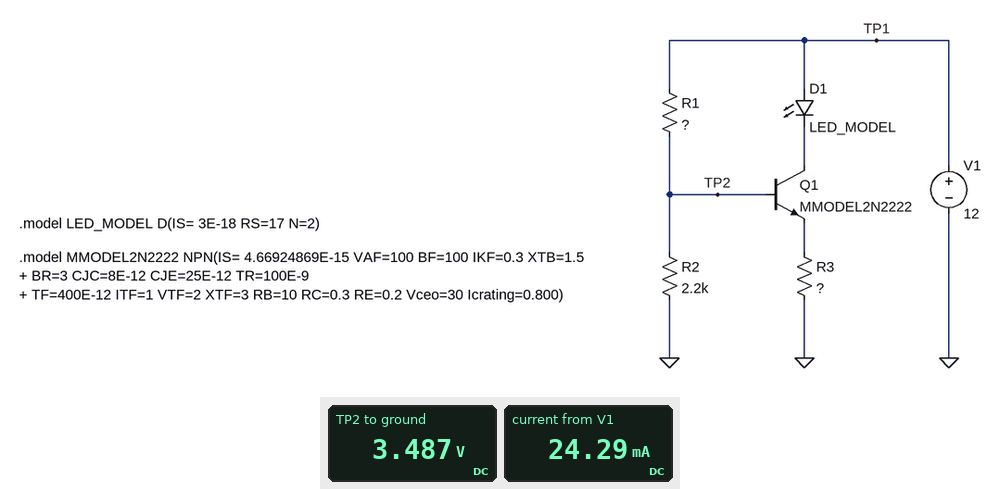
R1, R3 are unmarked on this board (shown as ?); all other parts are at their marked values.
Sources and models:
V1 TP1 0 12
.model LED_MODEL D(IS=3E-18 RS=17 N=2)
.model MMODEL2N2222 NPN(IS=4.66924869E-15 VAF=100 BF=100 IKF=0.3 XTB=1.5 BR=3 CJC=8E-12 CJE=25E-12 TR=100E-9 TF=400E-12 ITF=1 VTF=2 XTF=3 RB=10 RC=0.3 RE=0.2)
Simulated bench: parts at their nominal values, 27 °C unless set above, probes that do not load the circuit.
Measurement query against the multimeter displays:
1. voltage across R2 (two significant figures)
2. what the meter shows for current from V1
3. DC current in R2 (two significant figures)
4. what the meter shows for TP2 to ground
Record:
3.5 V
24.29 mA
1.6 mA
3.487 V
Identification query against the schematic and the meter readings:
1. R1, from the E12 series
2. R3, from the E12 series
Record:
4.7 kΩ
120 Ω
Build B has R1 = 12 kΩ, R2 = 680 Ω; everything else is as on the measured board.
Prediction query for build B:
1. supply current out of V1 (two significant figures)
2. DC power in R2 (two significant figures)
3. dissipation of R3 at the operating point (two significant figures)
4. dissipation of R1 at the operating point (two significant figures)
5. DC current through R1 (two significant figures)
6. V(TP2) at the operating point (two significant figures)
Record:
1.1 mA
610 µW
2.9 µW
11 mW
950 µA
640 mV
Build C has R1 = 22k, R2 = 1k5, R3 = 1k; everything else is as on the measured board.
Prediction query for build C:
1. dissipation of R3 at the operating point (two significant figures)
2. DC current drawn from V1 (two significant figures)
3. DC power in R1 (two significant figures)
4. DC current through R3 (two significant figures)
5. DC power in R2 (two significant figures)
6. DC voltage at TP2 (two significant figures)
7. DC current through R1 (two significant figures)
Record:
20 µW
650 µA
5.7 mW
140 µA
390 µW
760 mV
510 µA
